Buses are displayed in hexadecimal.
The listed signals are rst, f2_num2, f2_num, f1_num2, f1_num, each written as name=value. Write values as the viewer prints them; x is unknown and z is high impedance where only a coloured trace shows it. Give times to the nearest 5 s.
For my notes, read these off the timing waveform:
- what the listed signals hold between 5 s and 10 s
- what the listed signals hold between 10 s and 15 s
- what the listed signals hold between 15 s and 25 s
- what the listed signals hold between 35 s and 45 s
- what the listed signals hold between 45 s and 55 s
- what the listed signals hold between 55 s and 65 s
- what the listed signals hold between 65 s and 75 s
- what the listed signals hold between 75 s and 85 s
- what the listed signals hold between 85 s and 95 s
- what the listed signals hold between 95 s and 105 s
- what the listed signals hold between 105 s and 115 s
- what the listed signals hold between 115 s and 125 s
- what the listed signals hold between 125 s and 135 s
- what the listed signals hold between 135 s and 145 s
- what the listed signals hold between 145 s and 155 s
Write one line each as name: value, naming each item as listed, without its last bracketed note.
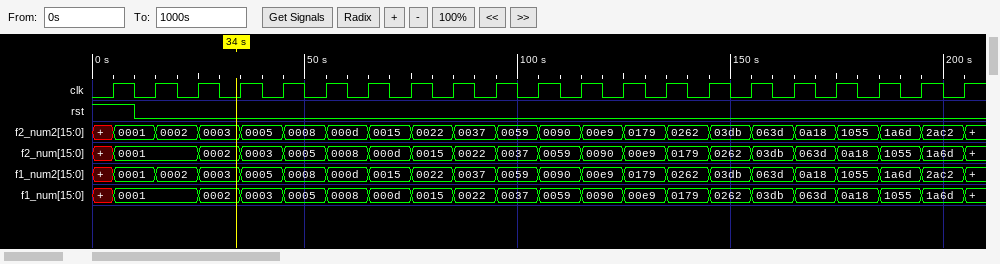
what the listed signals hold between 5 s and 10 s: rst=1, f2_num2=0001, f2_num=0001, f1_num2=0001, f1_num=0001
what the listed signals hold between 10 s and 15 s: rst=0, f2_num2=0001, f2_num=0001, f1_num2=0001, f1_num=0001
what the listed signals hold between 15 s and 25 s: rst=0, f2_num2=0002, f2_num=0001, f1_num2=0002, f1_num=0001
what the listed signals hold between 35 s and 45 s: rst=0, f2_num2=0005, f2_num=0003, f1_num2=0005, f1_num=0003
what the listed signals hold between 45 s and 55 s: rst=0, f2_num2=0008, f2_num=0005, f1_num2=0008, f1_num=0005
what the listed signals hold between 55 s and 65 s: rst=0, f2_num2=000d, f2_num=0008, f1_num2=000d, f1_num=0008
what the listed signals hold between 65 s and 75 s: rst=0, f2_num2=0015, f2_num=000d, f1_num2=0015, f1_num=000d
what the listed signals hold between 75 s and 85 s: rst=0, f2_num2=0022, f2_num=0015, f1_num2=0022, f1_num=0015
what the listed signals hold between 85 s and 95 s: rst=0, f2_num2=0037, f2_num=0022, f1_num2=0037, f1_num=0022
what the listed signals hold between 95 s and 105 s: rst=0, f2_num2=0059, f2_num=0037, f1_num2=0059, f1_num=0037
what the listed signals hold between 105 s and 115 s: rst=0, f2_num2=0090, f2_num=0059, f1_num2=0090, f1_num=0059
what the listed signals hold between 115 s and 125 s: rst=0, f2_num2=00e9, f2_num=0090, f1_num2=00e9, f1_num=0090
what the listed signals hold between 125 s and 135 s: rst=0, f2_num2=0179, f2_num=00e9, f1_num2=0179, f1_num=00e9
what the listed signals hold between 135 s and 145 s: rst=0, f2_num2=0262, f2_num=0179, f1_num2=0262, f1_num=0179
what the listed signals hold between 145 s and 155 s: rst=0, f2_num2=03db, f2_num=0262, f1_num2=03db, f1_num=0262
